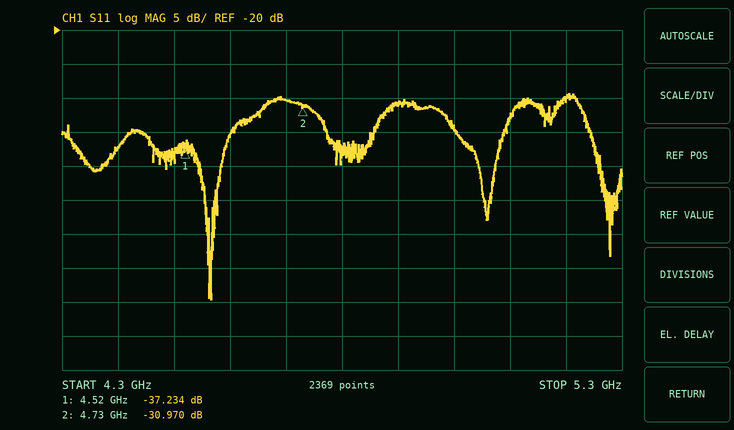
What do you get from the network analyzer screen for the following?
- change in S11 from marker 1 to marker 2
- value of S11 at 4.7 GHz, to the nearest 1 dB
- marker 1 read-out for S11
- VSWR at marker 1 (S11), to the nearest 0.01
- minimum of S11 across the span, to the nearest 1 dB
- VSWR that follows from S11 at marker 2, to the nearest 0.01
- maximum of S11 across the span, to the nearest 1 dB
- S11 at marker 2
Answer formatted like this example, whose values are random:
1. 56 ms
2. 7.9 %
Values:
1. 6.264 dB
2. -30 dB
3. -37.234 dB
4. 1.03
5. -60 dB
6. 1.06
7. -29 dB
8. -30.970 dB
